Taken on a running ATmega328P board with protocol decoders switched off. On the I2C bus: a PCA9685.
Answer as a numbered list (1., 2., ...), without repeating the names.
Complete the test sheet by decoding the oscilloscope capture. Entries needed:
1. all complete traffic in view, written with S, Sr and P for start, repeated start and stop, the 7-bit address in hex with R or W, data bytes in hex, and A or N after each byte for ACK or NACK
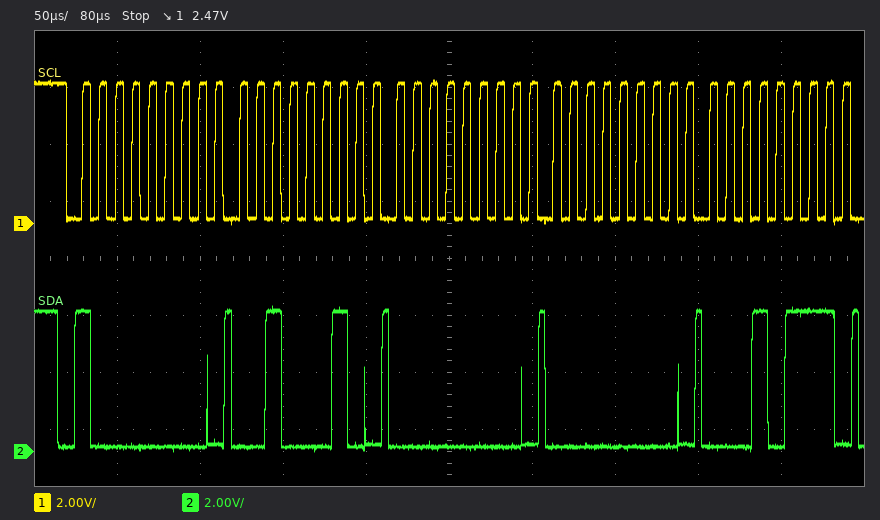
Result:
1. S 40W A 22 A 00 A 00 A 17 A
